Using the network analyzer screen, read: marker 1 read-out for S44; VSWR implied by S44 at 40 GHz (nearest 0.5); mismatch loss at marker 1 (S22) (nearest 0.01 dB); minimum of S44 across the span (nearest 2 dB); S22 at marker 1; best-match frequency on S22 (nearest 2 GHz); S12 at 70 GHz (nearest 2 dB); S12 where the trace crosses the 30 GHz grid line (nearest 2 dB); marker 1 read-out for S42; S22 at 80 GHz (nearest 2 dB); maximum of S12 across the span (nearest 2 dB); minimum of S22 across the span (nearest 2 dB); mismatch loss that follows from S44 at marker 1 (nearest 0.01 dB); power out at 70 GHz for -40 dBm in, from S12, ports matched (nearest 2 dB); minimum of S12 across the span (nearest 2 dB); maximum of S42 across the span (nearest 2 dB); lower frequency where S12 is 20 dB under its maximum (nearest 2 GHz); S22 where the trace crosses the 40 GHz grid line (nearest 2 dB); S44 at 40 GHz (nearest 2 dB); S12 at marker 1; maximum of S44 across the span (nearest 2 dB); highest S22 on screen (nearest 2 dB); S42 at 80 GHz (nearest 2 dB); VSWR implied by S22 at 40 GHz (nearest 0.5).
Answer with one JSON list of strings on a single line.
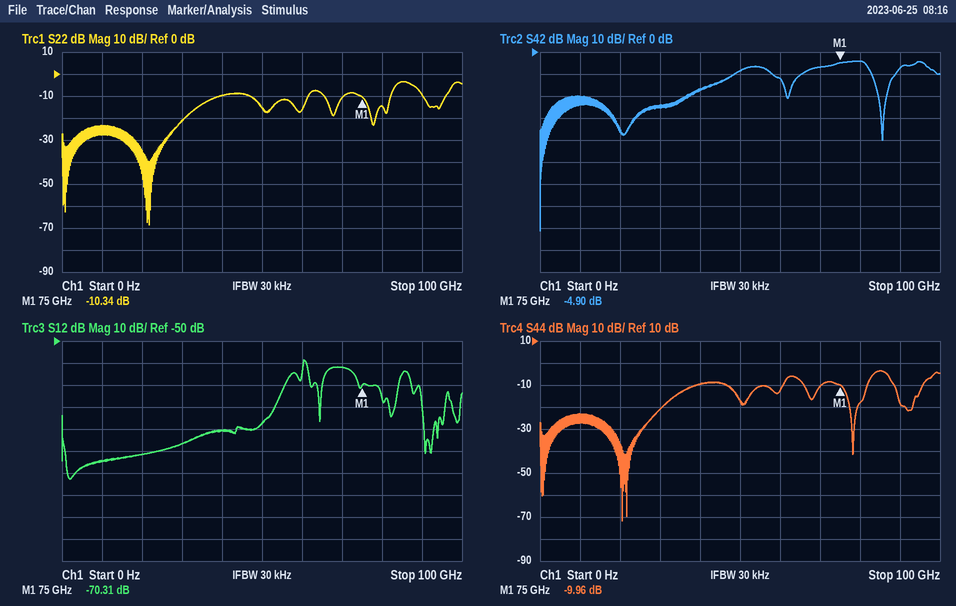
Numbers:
["-9.96 dB", "2.0", "0.42 dB", "-72 dB", "-10.34 dB", "22 GHz", "-62 dB", "-96 dB", "-4.90 dB", "-14 dB", "-58 dB", "-68 dB", "0.46 dB", "-102 dBm", "-112 dB", "-4 dB", "54 GHz", "-10 dB", "-10 dB", "-70.31 dB", "-4 dB", "-4 dB", "-4 dB", "2.0"]
